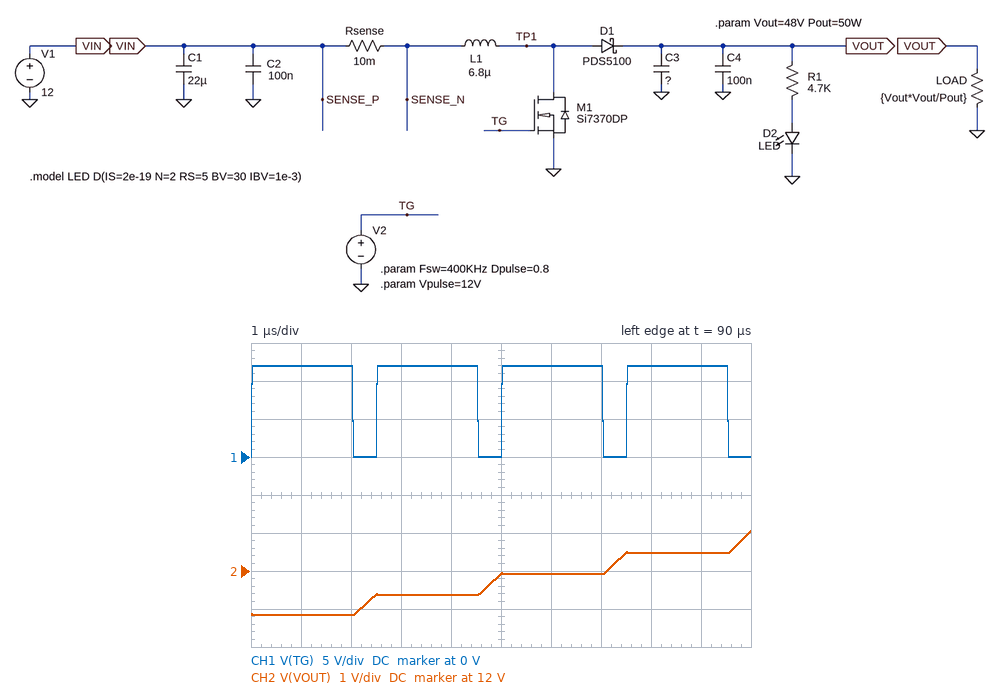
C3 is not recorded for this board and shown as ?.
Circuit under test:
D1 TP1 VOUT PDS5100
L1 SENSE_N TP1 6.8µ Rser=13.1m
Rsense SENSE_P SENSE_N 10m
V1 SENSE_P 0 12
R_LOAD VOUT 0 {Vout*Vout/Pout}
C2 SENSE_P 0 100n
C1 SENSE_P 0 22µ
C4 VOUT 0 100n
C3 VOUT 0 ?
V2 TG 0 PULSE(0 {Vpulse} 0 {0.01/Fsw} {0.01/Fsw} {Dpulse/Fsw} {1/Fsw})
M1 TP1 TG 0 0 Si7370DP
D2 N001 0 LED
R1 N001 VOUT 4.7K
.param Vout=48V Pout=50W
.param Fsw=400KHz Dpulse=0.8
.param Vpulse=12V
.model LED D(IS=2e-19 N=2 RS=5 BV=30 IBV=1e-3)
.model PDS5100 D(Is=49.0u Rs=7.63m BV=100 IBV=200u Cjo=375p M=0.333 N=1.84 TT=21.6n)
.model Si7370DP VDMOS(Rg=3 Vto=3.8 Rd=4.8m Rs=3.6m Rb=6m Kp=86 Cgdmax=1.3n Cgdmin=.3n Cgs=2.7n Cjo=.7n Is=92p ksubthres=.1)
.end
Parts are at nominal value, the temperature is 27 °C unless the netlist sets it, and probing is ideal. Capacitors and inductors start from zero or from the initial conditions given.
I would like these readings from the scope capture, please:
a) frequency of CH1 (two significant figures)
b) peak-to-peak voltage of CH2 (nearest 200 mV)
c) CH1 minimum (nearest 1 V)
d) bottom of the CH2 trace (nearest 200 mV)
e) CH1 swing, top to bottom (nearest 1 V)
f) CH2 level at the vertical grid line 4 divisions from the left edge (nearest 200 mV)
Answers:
400 kHz
2.2 V
0 V
10.8 V
12 V
11.4 V
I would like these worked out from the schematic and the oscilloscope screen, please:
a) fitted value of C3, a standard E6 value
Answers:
100 µF
